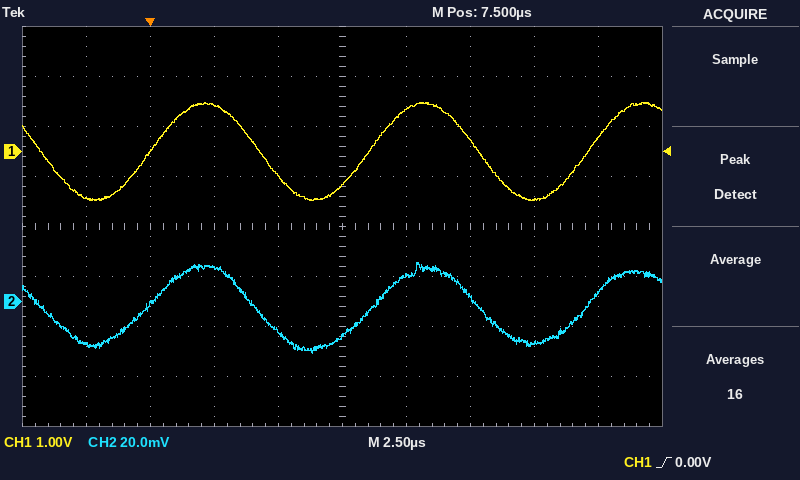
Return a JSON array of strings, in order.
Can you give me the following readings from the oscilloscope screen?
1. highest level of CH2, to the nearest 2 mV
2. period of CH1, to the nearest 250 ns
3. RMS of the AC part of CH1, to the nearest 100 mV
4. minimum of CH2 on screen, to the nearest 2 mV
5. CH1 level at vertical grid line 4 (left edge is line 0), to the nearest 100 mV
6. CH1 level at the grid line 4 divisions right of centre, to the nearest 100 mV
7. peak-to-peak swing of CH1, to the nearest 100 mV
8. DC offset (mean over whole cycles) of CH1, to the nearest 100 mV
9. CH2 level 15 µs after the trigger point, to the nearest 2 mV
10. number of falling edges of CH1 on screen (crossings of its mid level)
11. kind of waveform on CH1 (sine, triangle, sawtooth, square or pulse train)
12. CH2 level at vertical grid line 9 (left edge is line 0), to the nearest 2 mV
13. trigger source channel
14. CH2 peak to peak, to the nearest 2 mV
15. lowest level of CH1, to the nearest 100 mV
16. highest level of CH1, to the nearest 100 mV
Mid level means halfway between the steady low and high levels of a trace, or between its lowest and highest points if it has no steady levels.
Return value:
["16 mV", "8.50 µs", "700 mV", "-20 mV", "-500 mV", "300 mV", "2.0 V", "0.0 V", "-16 mV", "3", "sine", "4 mV", "CH1", "36 mV", "-1.0 V", "1.0 V"]
